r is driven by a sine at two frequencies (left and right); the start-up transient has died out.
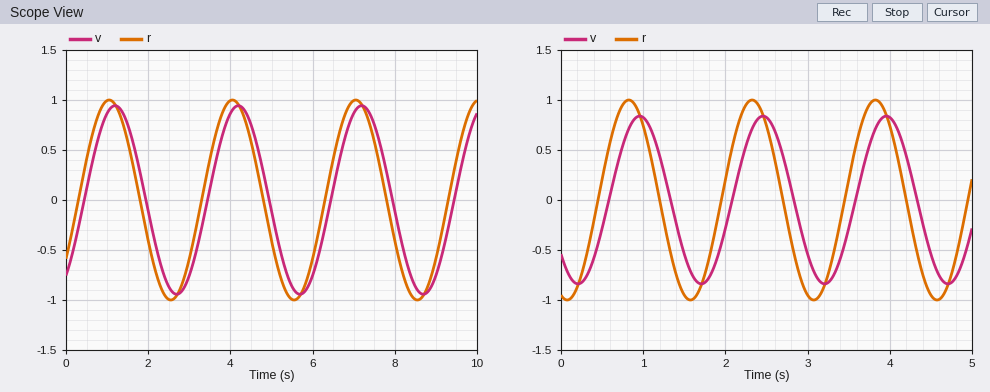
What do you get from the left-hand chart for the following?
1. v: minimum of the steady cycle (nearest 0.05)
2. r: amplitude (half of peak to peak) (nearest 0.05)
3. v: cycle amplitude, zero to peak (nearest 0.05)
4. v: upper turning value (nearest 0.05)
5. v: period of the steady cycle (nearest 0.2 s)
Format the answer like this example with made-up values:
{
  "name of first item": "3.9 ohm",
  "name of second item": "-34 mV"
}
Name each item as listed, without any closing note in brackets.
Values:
{
  "v: minimum of the steady cycle": "-0.95",
  "r: amplitude (half of peak to peak)": "1.00",
  "v: cycle amplitude, zero to peak": "0.95",
  "v: upper turning value": "0.95",
  "v: period of the steady cycle": "3.0 s"
}
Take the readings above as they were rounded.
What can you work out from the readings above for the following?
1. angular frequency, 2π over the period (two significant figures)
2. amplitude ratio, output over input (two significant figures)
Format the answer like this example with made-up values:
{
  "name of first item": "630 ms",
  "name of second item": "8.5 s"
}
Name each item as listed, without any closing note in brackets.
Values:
{
  "angular frequency, 2π over the period": "2.1 rad/s",
  "amplitude ratio, output over input": "0.95"
}
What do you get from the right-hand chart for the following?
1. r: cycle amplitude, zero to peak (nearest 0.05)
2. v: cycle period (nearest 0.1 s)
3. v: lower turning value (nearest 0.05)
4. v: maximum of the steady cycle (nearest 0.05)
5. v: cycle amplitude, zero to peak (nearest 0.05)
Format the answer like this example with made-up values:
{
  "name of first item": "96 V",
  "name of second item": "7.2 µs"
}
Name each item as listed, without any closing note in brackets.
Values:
{
  "r: cycle amplitude, zero to peak": "1.00",
  "v: cycle period": "1.5 s",
  "v: lower turning value": "-0.85",
  "v: maximum of the steady cycle": "0.85",
  "v: cycle amplitude, zero to peak": "0.85"
}
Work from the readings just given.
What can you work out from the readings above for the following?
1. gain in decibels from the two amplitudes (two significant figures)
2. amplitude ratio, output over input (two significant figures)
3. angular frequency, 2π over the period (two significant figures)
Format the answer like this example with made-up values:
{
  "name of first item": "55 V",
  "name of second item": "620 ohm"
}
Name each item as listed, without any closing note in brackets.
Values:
{
  "gain in decibels from the two amplitudes": "-1.4 dB",
  "amplitude ratio, output over input": "0.85",
  "angular frequency, 2π over the period": "4.2 rad/s"
}
